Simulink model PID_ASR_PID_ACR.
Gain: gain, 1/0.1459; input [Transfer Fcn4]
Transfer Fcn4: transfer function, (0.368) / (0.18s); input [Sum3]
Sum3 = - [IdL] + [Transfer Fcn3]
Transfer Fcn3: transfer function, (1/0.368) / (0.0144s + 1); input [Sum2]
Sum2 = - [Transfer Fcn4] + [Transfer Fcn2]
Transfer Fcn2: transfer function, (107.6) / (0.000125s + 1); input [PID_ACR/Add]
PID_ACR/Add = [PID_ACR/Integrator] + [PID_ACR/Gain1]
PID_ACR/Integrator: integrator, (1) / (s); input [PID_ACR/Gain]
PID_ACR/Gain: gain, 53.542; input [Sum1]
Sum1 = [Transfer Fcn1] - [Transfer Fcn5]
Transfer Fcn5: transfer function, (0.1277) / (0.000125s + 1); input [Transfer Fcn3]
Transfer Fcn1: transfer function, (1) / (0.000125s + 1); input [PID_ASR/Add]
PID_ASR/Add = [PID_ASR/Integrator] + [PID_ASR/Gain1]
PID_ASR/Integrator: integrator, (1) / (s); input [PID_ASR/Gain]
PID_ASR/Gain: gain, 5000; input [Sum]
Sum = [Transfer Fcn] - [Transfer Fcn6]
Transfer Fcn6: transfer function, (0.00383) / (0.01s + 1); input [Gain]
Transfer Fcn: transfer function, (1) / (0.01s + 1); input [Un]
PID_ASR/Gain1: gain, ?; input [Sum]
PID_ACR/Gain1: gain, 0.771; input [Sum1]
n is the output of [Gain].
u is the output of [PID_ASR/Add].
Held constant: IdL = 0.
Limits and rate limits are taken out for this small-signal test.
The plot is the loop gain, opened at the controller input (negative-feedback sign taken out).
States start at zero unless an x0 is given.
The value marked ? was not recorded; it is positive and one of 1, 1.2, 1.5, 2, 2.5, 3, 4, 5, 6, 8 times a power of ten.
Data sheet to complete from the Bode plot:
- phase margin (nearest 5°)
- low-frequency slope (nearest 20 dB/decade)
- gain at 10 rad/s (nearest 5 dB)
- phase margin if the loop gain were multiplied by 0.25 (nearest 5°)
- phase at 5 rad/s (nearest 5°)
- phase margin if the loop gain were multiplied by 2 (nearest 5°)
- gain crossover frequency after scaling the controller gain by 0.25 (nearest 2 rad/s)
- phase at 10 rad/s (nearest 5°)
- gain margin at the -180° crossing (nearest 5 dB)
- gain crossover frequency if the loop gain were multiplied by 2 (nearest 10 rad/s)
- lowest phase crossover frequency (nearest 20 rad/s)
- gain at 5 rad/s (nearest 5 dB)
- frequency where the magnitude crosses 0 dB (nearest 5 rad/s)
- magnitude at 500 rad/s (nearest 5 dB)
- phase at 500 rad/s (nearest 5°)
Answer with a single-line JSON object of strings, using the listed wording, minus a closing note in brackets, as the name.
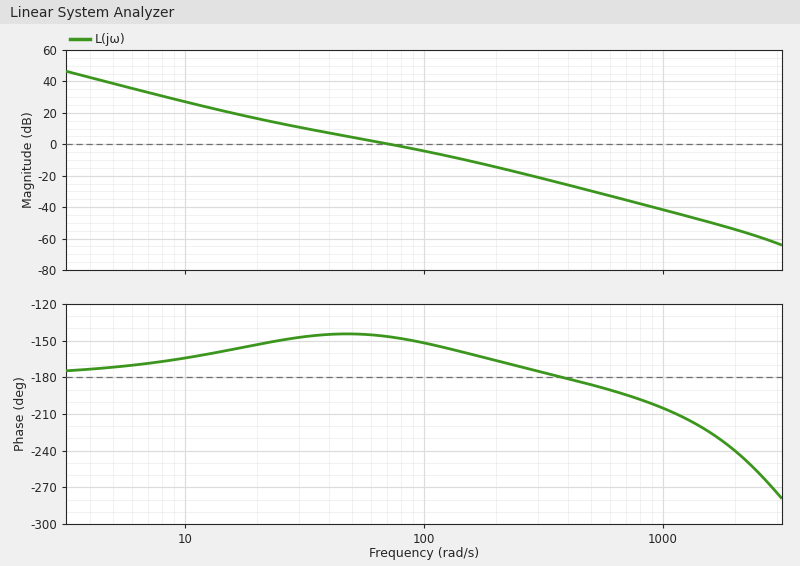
{"phase margin": "35°", "low-frequency slope": "-40 dB/decade", "gain at 10 rad/s": "25 dB", "phase margin if the loop gain were multiplied by 0.25": "30°", "phase at 5 rad/s": "-170°", "phase margin if the loop gain were multiplied by 2": "25°", "gain crossover frequency after scaling the controller gain by 0.25": "28 rad/s", "phase at 10 rad/s": "-165°", "gain margin at the -180° crossing": "25 dB", "gain crossover frequency if the loop gain were multiplied by 2": "110 rad/s", "lowest phase crossover frequency": "380 rad/s", "gain at 5 rad/s": "40 dB", "frequency where the magnitude crosses 0 dB": "70 rad/s", "magnitude at 500 rad/s": "-30 dB", "phase at 500 rad/s": "-185°"}
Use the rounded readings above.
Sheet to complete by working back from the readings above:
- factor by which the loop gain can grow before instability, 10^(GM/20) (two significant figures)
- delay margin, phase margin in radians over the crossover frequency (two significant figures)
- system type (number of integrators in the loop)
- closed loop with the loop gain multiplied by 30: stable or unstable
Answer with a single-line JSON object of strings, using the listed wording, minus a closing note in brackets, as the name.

{"factor by which the loop gain can grow before instability, 10^(GM/20)": "18", "delay margin, phase margin in radians over the crossover frequency": "0.0087 s", "system type": "2", "closed loop with the loop gain multiplied by 30: stable or unstable": "unstable"}
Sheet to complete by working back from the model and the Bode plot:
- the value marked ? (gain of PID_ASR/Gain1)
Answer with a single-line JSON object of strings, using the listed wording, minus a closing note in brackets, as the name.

{"the value marked ?": "200"}
